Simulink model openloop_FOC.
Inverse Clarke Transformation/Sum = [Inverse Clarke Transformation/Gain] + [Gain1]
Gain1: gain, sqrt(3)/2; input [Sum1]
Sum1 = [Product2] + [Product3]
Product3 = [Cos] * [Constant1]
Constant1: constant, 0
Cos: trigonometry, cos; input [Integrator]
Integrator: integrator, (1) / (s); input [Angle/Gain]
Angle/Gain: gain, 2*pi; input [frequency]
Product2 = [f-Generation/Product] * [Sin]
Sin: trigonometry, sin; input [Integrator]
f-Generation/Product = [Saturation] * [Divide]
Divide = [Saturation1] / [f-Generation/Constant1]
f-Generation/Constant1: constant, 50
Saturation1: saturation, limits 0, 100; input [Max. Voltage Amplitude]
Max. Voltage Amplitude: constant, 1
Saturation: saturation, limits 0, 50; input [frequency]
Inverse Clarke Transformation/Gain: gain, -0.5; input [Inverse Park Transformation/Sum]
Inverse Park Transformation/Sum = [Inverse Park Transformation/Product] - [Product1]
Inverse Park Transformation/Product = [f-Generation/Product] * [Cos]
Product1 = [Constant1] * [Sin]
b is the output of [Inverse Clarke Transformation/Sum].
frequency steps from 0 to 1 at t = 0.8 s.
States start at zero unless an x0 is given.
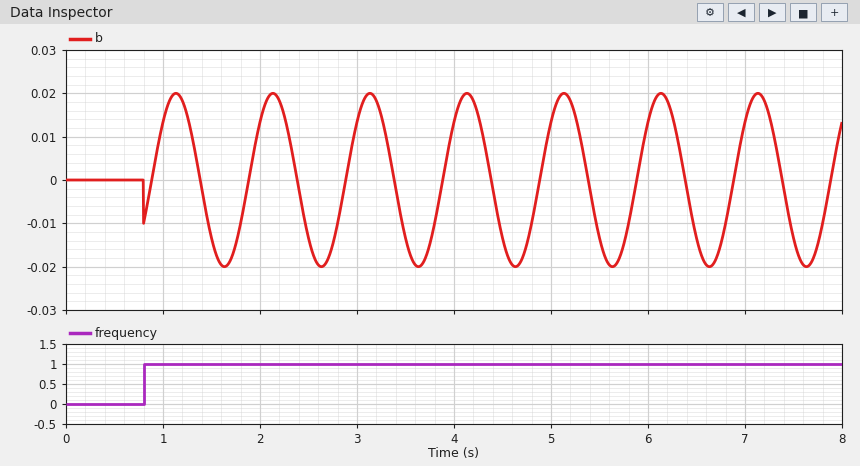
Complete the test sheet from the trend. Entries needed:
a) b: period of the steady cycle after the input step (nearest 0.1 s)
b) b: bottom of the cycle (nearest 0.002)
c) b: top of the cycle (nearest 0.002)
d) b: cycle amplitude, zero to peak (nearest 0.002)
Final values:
1.0 s
-0.020
0.020
0.020
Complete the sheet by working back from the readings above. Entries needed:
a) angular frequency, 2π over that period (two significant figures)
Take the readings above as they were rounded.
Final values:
6.3 rad/s
